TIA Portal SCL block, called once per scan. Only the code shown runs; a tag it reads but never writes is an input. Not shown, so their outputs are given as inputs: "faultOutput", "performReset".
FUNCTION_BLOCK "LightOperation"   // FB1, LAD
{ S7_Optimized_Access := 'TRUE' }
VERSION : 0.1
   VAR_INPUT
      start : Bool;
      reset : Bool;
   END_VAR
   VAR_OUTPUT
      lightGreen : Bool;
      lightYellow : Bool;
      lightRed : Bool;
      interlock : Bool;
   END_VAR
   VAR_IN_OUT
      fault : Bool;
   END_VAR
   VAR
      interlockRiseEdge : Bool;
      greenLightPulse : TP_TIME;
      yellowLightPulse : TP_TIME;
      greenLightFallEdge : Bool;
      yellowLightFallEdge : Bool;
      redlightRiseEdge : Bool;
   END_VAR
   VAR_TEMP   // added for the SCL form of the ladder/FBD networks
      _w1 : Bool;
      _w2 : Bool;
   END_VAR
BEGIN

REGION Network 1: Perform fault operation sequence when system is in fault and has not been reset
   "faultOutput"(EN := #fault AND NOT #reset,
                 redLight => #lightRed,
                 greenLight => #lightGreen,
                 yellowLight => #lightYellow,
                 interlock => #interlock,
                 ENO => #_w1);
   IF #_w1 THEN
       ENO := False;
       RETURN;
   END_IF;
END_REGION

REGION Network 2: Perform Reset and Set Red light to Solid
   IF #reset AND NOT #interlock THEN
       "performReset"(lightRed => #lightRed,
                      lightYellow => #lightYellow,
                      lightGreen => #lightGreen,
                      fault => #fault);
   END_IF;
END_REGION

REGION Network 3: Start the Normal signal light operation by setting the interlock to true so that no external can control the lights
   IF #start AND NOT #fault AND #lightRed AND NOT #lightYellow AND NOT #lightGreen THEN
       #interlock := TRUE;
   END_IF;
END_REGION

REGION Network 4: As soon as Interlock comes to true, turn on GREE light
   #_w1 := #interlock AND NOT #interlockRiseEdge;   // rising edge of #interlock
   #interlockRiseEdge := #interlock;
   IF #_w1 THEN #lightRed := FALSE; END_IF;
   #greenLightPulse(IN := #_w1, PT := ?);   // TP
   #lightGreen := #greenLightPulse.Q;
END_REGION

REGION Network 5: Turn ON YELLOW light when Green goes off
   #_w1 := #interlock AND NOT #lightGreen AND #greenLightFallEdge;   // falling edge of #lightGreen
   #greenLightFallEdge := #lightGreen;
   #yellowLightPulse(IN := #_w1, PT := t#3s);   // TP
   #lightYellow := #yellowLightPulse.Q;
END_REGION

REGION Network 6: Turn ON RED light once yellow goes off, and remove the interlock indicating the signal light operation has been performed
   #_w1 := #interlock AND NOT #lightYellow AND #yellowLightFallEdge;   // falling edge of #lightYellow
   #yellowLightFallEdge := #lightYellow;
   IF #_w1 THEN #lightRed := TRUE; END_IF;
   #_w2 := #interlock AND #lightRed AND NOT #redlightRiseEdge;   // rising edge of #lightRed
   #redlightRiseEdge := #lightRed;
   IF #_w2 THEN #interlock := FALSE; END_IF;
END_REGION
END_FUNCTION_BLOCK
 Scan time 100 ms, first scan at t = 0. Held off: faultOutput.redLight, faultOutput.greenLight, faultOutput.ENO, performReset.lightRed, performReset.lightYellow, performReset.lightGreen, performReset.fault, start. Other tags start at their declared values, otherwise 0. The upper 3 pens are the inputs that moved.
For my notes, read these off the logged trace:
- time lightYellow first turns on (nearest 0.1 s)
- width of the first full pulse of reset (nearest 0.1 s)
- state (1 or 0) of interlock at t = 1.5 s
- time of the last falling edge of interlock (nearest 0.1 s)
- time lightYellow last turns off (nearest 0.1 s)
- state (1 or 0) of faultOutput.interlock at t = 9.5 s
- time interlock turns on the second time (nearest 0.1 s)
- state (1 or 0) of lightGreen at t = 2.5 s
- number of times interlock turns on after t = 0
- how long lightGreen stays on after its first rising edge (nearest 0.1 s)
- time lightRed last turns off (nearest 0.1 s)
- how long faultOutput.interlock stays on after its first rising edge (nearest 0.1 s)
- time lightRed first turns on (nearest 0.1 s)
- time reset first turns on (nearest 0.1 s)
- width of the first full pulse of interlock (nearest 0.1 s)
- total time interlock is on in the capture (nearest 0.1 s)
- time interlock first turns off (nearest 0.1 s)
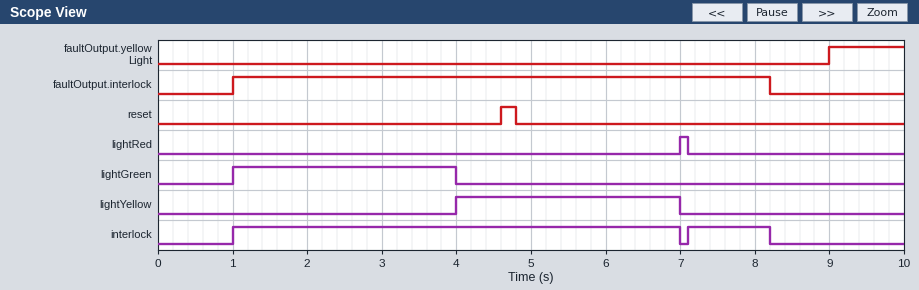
4.0 s
0.2 s
1
8.2 s
7.0 s
0
7.1 s
1
2
3.0 s
7.1 s
7.2 s
7.0 s
4.6 s
6.0 s
7.1 s
7.0 s
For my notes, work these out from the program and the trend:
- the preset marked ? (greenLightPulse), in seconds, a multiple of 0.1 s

3.0 s
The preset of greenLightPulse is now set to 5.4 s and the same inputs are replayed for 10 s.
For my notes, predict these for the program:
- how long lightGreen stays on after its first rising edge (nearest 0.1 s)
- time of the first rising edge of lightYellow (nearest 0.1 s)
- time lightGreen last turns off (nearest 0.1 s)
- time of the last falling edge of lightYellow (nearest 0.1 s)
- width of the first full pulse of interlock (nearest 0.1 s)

5.4 s
6.4 s
6.4 s
9.4 s
7.2 s
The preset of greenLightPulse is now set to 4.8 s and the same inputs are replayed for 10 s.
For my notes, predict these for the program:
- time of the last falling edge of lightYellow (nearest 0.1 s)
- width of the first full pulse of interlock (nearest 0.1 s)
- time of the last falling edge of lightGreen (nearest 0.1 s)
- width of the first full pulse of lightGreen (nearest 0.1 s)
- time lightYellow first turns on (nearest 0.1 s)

8.8 s
7.2 s
5.8 s
4.8 s
5.8 s
